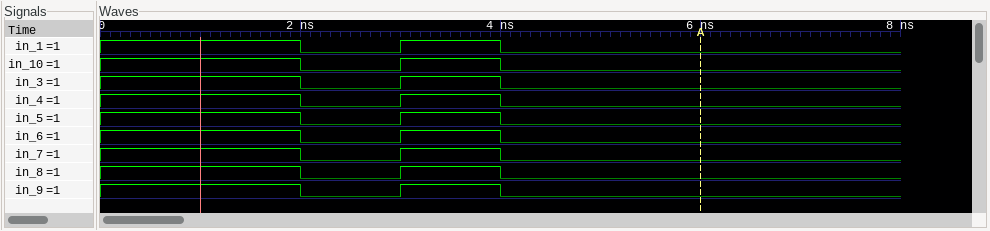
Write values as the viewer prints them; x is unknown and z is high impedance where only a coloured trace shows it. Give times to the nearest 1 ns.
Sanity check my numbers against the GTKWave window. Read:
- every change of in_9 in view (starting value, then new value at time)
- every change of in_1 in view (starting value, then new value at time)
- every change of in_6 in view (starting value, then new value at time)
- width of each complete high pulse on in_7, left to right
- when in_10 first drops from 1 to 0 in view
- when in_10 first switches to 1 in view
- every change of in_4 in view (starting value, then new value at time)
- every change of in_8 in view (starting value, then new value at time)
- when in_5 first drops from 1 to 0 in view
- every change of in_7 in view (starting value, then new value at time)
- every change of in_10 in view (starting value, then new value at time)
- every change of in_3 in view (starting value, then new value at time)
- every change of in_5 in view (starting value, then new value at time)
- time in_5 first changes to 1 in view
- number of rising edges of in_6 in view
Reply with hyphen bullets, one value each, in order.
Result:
- 1, 0 at 2 ns, 1 at 3 ns, 0 at 4 ns
- 1, 0 at 2 ns, 1 at 3 ns, 0 at 4 ns
- 1, 0 at 2 ns, 1 at 3 ns, 0 at 4 ns
- 1 ns
- 2 ns
- 3 ns
- 1, 0 at 2 ns, 1 at 3 ns, 0 at 4 ns
- 1, 0 at 2 ns, 1 at 3 ns, 0 at 4 ns
- 2 ns
- 1, 0 at 2 ns, 1 at 3 ns, 0 at 4 ns
- 1, 0 at 2 ns, 1 at 3 ns, 0 at 4 ns
- 1, 0 at 2 ns, 1 at 3 ns, 0 at 4 ns
- 1, 0 at 2 ns, 1 at 3 ns, 0 at 4 ns
- 3 ns
- 1
